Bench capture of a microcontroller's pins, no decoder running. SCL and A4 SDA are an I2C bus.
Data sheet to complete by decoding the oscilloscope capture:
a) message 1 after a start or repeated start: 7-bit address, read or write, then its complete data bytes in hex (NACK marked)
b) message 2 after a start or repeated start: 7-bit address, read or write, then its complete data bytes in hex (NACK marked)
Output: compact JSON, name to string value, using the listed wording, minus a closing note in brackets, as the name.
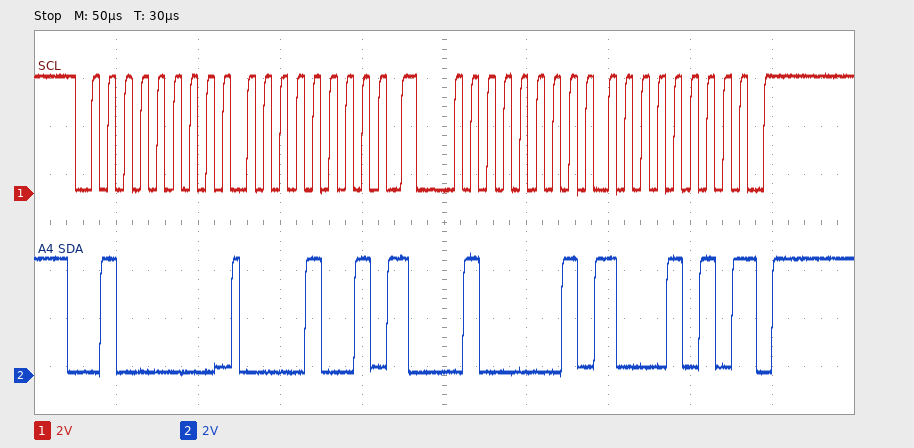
{"message 1 after a start or repeated start: 7-bit address, read or write, then its complete data bytes in hex": "0x20 write: 09", "message 2 after a start or repeated start: 7-bit address, read or write, then its complete data bytes in hex": "0x20 read: 8A NACK"}
